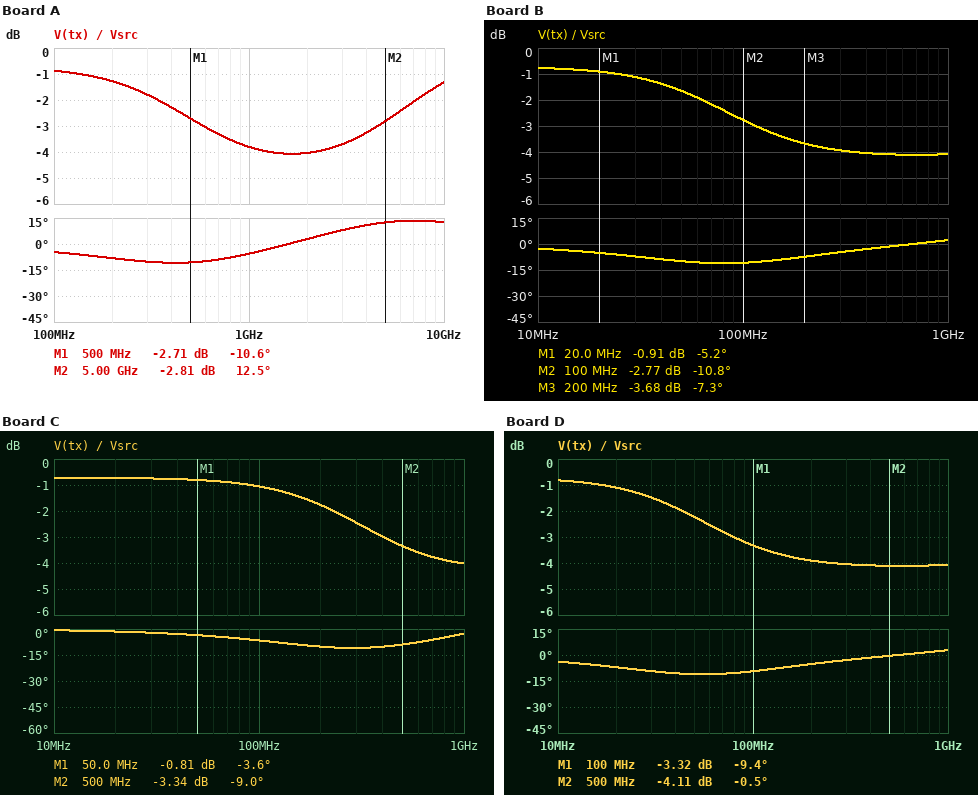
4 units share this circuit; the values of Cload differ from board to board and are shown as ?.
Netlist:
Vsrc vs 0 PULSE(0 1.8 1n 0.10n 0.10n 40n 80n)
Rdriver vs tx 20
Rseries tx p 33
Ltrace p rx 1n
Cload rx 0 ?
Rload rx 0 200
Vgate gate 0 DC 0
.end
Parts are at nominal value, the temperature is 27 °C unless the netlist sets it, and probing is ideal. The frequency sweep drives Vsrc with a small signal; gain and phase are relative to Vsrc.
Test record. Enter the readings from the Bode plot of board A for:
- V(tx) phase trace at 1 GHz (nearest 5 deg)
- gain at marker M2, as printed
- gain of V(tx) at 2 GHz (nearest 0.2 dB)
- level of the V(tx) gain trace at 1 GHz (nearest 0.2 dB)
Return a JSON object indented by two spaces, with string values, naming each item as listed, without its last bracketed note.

{
  "V(tx) phase trace at 1 GHz": "-5 deg",
  "gain at marker M2, as printed": "-2.81 dB",
  "gain of V(tx) at 2 GHz": "-4.0 dB",
  "level of the V(tx) gain trace at 1 GHz": "-3.8 dB"
}
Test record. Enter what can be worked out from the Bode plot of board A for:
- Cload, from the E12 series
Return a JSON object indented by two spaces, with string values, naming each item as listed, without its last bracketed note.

{
  "Cload, from the E12 series": "10 pF"
}
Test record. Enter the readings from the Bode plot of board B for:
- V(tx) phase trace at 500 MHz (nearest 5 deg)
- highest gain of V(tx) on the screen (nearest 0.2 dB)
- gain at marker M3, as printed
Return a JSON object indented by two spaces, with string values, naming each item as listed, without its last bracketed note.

{
  "V(tx) phase trace at 500 MHz": "0 deg",
  "highest gain of V(tx) on the screen": "-0.8 dB",
  "gain at marker M3, as printed": "-3.68 dB"
}
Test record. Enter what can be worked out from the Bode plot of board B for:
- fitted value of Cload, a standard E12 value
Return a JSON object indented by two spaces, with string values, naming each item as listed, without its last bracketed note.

{
  "fitted value of Cload, a standard E12 value": "56 pF"
}
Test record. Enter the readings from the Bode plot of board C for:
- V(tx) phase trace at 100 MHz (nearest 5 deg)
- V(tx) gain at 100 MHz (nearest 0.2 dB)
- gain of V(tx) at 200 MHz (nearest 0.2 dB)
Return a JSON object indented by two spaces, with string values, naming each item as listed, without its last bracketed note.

{
  "V(tx) phase trace at 100 MHz": "-5 deg",
  "V(tx) gain at 100 MHz": "-1.0 dB",
  "gain of V(tx) at 200 MHz": "-1.8 dB"
}
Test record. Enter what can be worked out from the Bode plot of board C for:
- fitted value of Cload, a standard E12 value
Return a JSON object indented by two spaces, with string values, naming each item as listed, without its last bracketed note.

{
  "fitted value of Cload, a standard E12 value": "15 pF"
}
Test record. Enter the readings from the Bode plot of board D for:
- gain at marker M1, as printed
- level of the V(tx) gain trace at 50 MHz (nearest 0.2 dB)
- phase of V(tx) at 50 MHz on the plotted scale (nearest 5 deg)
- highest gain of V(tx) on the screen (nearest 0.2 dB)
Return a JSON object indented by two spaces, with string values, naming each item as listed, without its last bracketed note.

{
  "gain at marker M1, as printed": "-3.32 dB",
  "level of the V(tx) gain trace at 50 MHz": "-2.2 dB",
  "phase of V(tx) at 50 MHz on the plotted scale": "-10 deg",
  "highest gain of V(tx) on the screen": "-0.8 dB"
}
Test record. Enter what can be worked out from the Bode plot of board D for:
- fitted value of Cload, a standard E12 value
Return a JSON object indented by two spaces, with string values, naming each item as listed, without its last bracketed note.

{
  "fitted value of Cload, a standard E12 value": "82 pF"
}
